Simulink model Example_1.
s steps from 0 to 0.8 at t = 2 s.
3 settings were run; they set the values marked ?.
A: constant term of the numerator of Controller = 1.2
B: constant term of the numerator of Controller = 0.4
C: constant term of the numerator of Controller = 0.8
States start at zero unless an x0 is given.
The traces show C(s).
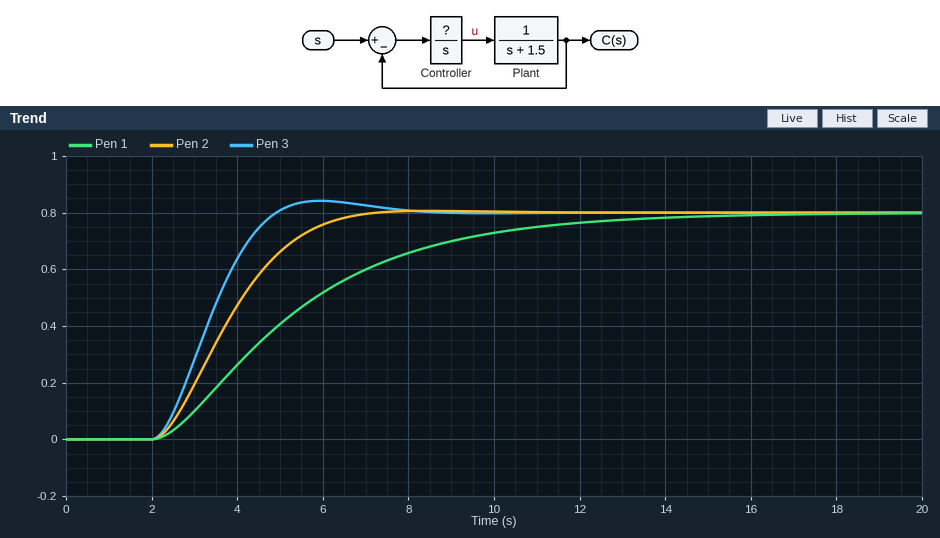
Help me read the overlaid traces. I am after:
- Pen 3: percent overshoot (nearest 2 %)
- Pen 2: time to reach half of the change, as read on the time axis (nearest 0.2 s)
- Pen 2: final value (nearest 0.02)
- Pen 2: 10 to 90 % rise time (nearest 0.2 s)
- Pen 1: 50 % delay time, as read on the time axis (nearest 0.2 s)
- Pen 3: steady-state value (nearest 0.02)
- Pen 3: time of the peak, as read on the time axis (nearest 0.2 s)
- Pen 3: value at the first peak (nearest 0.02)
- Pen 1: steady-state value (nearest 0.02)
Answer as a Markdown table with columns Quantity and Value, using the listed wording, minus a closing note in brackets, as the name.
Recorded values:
| Quantity | Value |
|---|---|
| Pen 3: percent overshoot | 6 % |
| Pen 2: time to reach half of the change, as read on the time axis | 3.8 s |
| Pen 2: final value | 0.80 |
| Pen 2: 10 to 90 % rise time | 3.0 s |
| Pen 1: 50 % delay time, as read on the time axis | 5.0 s |
| Pen 3: steady-state value | 0.80 |
| Pen 3: time of the peak, as read on the time axis | 6.0 s |
| Pen 3: value at the first peak | 0.84 |
| Pen 1: steady-state value | 0.80 |
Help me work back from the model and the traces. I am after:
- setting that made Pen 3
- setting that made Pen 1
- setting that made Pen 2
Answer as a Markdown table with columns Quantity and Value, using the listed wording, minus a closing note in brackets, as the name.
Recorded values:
| Quantity | Value |
|---|---|
| setting that made Pen 3 | A |
| setting that made Pen 1 | B |
| setting that made Pen 2 | C |
